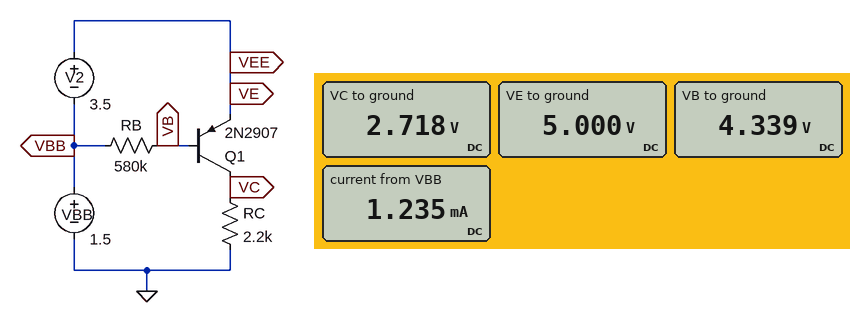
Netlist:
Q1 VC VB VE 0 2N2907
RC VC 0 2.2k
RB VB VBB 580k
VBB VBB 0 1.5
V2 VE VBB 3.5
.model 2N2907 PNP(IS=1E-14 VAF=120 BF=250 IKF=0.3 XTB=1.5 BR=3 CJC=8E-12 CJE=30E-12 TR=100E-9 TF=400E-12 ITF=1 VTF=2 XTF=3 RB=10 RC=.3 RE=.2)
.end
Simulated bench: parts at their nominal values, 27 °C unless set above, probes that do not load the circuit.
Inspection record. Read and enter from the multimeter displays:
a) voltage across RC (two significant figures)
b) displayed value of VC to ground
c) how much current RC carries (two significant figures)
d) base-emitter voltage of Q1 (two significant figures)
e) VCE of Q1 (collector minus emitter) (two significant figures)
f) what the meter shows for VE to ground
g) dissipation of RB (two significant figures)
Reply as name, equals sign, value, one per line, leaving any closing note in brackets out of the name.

voltage across RC = 2.7 V
displayed value of VC to ground = 2.718 V
how much current RC carries = 1.2 mA
base-emitter voltage of Q1 = -660 mV
VCE of Q1 (collector minus emitter) = -2.3 V
what the meter shows for VE to ground = 5.000 V
dissipation of RB = 14 µW
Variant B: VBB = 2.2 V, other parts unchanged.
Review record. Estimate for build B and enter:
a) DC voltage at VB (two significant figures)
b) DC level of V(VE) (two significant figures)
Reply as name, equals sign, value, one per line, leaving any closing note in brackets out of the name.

DC voltage at VB = 5.0 V
DC level of V(VE) = 5.7 V
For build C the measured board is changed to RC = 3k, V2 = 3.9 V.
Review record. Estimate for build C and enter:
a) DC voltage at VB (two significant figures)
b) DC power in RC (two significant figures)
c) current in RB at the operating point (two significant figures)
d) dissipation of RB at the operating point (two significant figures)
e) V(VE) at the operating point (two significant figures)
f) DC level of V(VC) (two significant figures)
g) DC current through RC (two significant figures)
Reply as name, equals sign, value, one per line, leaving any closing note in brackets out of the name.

DC voltage at VB = 4.7 V
DC power in RC = 5.8 mW
current in RB at the operating point = 5.6 µA
dissipation of RB at the operating point = 18 µW
V(VE) at the operating point = 5.4 V
DC level of V(VC) = 4.2 V
DC current through RC = 1.4 mA
